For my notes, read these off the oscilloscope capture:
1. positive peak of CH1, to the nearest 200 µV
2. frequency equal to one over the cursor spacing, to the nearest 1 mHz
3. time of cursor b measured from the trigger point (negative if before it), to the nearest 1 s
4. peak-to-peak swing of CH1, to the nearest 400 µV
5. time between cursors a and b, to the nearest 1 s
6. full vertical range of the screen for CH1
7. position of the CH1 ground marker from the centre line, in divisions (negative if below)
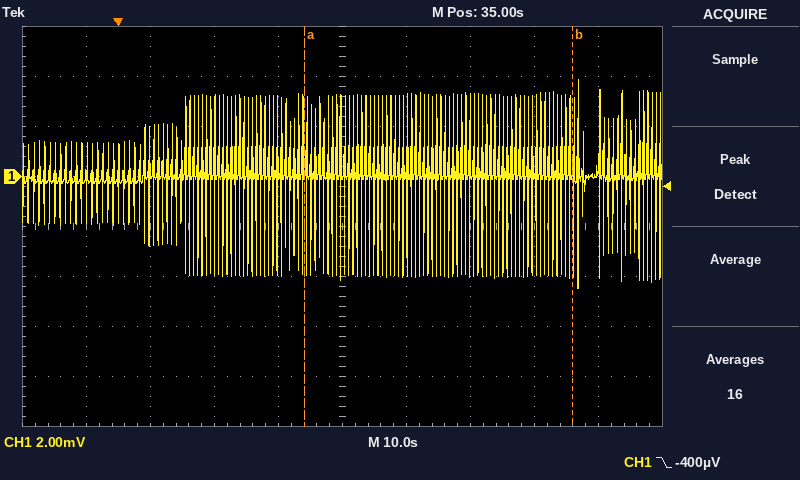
3.8 mV
24 mHz
+71 s
8.4 mV
42 s
16 mV
+1.0 div
